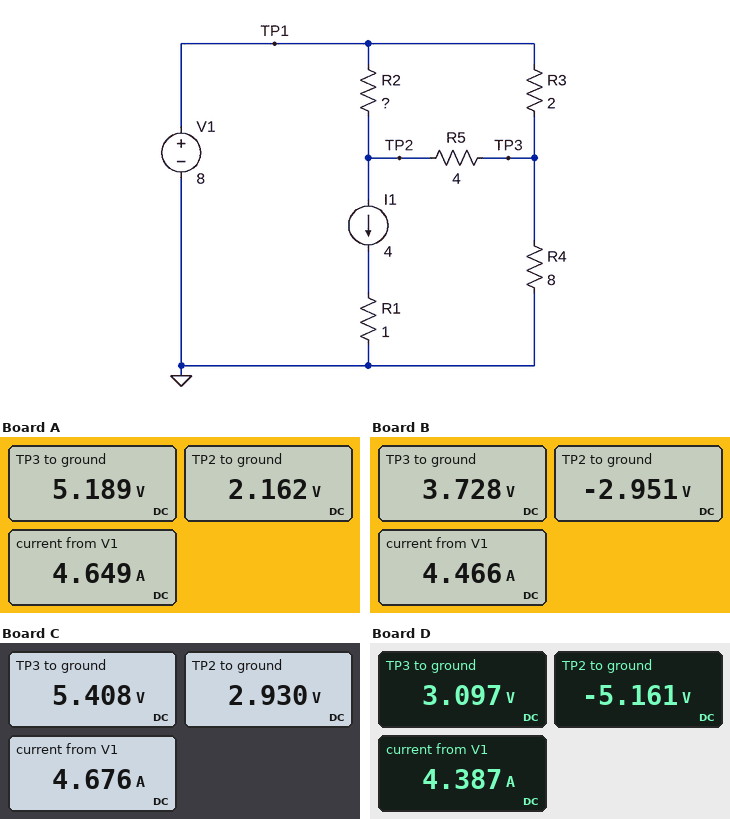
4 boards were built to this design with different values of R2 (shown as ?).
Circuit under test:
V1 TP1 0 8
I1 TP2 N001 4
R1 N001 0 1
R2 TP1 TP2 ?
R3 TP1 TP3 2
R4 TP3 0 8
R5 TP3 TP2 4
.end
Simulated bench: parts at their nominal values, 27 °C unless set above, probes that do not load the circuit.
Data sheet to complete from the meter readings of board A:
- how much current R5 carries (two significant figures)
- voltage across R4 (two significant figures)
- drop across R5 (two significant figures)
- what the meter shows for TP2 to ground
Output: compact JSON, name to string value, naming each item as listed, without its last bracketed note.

{"how much current R5 carries": "760 mA", "voltage across R4": "5.2 V", "drop across R5": "3.0 V", "what the meter shows for TP2 to ground": "2.162 V"}
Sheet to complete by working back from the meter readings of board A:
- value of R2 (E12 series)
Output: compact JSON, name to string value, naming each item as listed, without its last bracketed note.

{"value of R2": "1.8 Ω"}
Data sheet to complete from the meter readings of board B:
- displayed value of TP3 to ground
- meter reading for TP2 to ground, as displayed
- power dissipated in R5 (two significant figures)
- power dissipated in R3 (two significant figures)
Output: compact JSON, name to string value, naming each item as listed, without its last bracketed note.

{"displayed value of TP3 to ground": "3.728 V", "meter reading for TP2 to ground, as displayed": "-2.951 V", "power dissipated in R5": "11 W", "power dissipated in R3": "9.1 W"}
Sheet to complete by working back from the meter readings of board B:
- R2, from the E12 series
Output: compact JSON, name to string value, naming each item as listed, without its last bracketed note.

{"R2, from the E12 series": "4.7 Ω"}
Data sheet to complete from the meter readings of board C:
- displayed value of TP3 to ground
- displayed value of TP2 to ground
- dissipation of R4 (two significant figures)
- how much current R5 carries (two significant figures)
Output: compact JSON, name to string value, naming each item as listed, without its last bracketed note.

{"displayed value of TP3 to ground": "5.408 V", "displayed value of TP2 to ground": "2.930 V", "dissipation of R4": "3.7 W", "how much current R5 carries": "620 mA"}
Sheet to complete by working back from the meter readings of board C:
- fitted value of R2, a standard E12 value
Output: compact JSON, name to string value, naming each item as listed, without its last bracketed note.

{"fitted value of R2, a standard E12 value": "1.5 Ω"}
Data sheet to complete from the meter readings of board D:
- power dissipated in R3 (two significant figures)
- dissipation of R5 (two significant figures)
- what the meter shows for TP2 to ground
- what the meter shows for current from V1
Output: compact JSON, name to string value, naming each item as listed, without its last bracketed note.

{"power dissipated in R3": "12 W", "dissipation of R5": "17 W", "what the meter shows for TP2 to ground": "-5.161 V", "what the meter shows for current from V1": "4.387 A"}
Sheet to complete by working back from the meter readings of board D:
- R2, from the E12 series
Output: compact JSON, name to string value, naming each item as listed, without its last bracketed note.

{"R2, from the E12 series": "6.8 Ω"}
